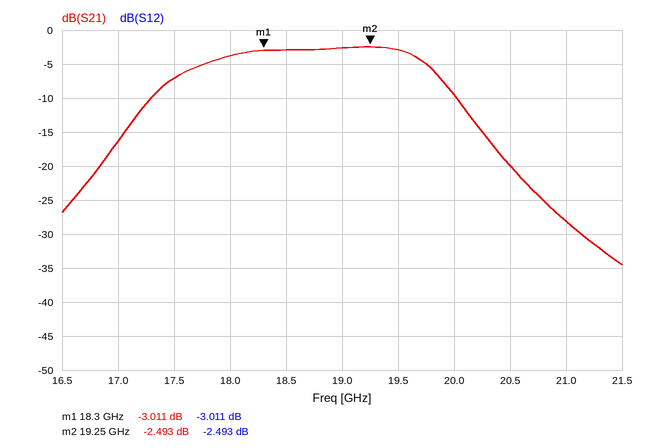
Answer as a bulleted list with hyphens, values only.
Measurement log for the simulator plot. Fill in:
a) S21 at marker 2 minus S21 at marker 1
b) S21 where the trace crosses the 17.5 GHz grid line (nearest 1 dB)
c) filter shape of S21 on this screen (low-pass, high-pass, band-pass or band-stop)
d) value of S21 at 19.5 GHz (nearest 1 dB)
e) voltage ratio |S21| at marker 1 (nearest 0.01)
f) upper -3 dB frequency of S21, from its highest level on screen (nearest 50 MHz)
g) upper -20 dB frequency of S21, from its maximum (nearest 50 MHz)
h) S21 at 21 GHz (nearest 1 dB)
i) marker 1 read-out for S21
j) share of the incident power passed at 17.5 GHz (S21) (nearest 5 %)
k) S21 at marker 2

- 0.518 dB
- -7 dB
- band-pass
- -3 dB
- 0.71
- 19.80 GHz
- 20.65 GHz
- -28 dB
- -3.011 dB
- 20 %
- -2.493 dB
